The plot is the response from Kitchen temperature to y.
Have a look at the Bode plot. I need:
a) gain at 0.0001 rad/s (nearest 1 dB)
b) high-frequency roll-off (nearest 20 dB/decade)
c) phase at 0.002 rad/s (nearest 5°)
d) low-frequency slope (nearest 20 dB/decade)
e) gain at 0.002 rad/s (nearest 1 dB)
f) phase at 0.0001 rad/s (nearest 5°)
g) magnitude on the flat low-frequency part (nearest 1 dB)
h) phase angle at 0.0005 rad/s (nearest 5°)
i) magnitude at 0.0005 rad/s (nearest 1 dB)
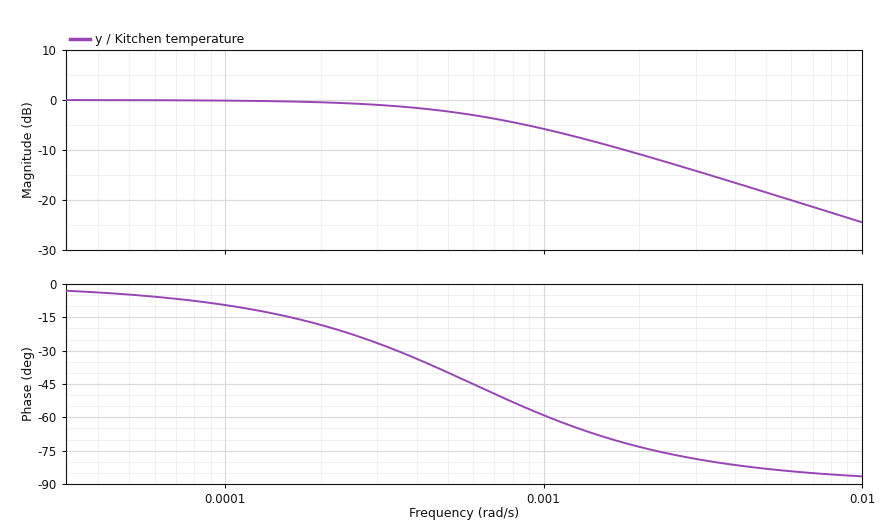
0 dB
-20 dB/decade
-75°
0 dB/decade
-11 dB
-10°
0 dB
-40°
-2 dB
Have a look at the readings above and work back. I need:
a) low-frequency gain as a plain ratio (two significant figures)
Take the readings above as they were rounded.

1.0
